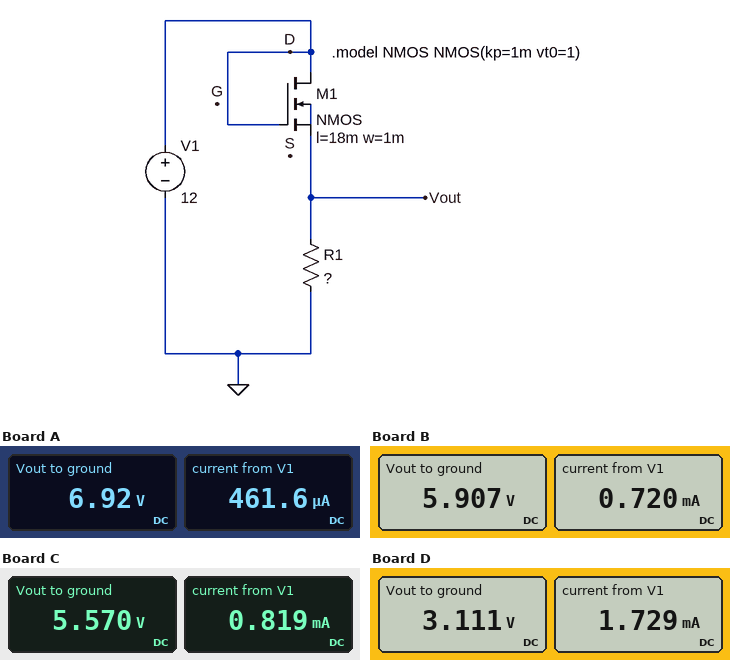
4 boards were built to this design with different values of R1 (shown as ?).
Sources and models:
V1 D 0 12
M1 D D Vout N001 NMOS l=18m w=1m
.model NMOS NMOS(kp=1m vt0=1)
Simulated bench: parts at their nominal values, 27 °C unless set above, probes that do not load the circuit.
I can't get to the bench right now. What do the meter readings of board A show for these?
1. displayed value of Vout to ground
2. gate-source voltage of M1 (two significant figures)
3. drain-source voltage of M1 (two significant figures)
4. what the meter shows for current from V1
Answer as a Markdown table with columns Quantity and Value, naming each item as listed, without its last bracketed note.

| Quantity | Value |
|---|---|
| displayed value of Vout to ground | 6.92 V |
| gate-source voltage of M1 | 5.1 V |
| drain-source voltage of M1 | 5.1 V |
| what the meter shows for current from V1 | 461.6 µA |
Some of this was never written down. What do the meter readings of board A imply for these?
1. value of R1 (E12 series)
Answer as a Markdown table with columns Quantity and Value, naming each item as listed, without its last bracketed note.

| Quantity | Value |
|---|---|
| value of R1 | 15 kΩ |
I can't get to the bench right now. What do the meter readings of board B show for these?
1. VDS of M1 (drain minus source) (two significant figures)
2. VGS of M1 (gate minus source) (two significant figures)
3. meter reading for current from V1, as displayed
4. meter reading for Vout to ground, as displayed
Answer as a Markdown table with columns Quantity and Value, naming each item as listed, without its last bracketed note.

| Quantity | Value |
|---|---|
| VDS of M1 (drain minus source) | 6.1 V |
| VGS of M1 (gate minus source) | 6.1 V |
| meter reading for current from V1, as displayed | 0.720 mA |
| meter reading for Vout to ground, as displayed | 5.907 V |
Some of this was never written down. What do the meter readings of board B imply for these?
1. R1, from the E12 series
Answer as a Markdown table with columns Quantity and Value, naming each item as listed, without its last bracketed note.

| Quantity | Value |
|---|---|
| R1, from the E12 series | 8.2 kΩ |
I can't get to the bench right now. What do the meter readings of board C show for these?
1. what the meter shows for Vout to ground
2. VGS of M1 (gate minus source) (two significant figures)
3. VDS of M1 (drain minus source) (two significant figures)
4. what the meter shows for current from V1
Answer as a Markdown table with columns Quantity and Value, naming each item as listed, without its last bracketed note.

| Quantity | Value |
|---|---|
| what the meter shows for Vout to ground | 5.570 V |
| VGS of M1 (gate minus source) | 6.4 V |
| VDS of M1 (drain minus source) | 6.4 V |
| what the meter shows for current from V1 | 0.819 mA |
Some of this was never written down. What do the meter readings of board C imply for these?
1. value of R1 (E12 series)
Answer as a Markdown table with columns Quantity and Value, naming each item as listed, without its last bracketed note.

| Quantity | Value |
|---|---|
| value of R1 | 6.8 kΩ |
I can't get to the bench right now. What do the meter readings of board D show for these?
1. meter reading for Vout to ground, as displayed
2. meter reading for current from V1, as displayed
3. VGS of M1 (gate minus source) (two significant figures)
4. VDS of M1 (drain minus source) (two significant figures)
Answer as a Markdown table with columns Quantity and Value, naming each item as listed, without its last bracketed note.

| Quantity | Value |
|---|---|
| meter reading for Vout to ground, as displayed | 3.111 V |
| meter reading for current from V1, as displayed | 1.729 mA |
| VGS of M1 (gate minus source) | 8.9 V |
| VDS of M1 (drain minus source) | 8.9 V |
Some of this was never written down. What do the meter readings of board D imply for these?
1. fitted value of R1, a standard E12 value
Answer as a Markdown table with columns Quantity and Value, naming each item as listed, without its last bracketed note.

| Quantity | Value |
|---|---|
| fitted value of R1, a standard E12 value | 1.8 kΩ |
